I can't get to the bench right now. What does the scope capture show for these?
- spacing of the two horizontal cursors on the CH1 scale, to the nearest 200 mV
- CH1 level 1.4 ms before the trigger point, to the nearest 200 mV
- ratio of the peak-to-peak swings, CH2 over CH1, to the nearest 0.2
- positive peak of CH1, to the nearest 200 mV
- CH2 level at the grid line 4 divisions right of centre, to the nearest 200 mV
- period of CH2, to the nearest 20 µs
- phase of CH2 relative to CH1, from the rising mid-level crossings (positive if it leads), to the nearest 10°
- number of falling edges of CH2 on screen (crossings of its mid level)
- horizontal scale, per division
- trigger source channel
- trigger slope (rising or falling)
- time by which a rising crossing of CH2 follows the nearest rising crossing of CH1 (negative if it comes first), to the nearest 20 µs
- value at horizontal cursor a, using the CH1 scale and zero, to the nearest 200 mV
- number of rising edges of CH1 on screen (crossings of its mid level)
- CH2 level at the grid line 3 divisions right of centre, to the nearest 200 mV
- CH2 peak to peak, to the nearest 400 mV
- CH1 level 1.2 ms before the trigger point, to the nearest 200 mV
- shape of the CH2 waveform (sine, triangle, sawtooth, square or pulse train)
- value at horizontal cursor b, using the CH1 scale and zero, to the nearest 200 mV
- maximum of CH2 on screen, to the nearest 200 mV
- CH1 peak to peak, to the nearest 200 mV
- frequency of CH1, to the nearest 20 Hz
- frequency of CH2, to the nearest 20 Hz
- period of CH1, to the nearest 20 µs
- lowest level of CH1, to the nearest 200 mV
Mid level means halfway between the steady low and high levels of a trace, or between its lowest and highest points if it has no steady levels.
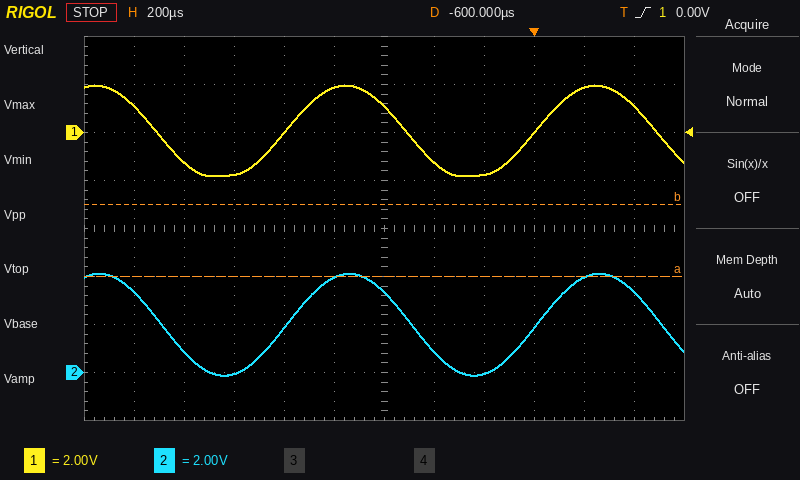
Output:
3.0 V
-1.2 V
1.2
2.0 V
4.0 V
1.00 ms
0°
3
200 µs
CH1
rising
0 µs
-6.0 V
2
1.8 V
4.4 V
-1.8 V
sine
-3.0 V
4.2 V
3.8 V
1.00 kHz
1.00 kHz
1.00 ms
-1.8 V
